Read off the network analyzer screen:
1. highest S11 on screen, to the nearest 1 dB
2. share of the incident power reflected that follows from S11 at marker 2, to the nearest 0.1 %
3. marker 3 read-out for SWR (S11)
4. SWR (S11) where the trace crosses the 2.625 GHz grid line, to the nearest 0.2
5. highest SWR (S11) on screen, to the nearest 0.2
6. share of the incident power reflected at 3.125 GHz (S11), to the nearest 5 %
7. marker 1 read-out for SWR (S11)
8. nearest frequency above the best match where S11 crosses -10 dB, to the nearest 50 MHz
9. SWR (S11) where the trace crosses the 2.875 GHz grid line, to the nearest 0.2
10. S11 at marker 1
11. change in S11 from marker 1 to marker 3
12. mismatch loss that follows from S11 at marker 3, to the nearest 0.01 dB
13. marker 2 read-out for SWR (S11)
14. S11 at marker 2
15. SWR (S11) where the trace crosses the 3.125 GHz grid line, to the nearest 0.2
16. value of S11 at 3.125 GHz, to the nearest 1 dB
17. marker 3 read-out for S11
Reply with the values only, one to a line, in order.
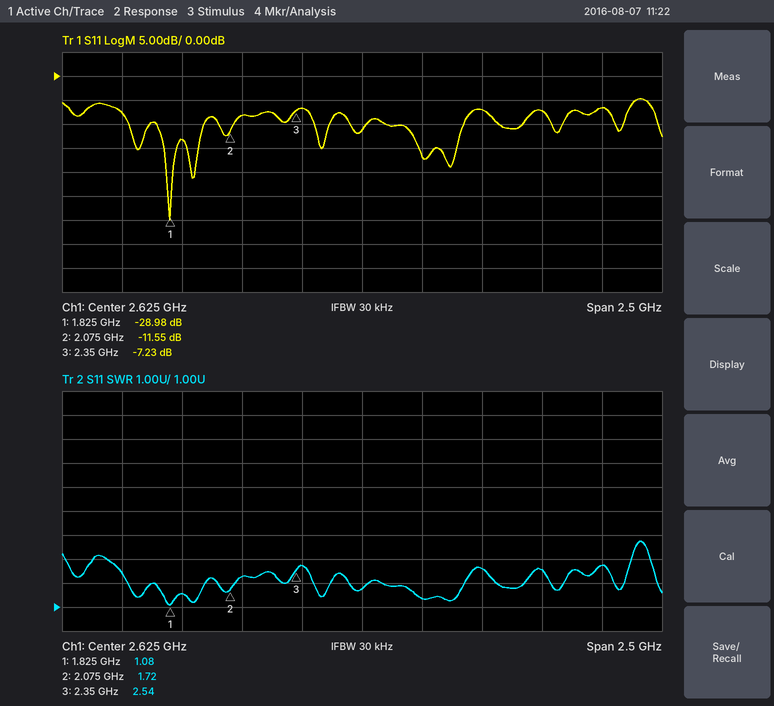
-5 dB
7.0 %
2.54
1.8
3.8
20 %
1.08
1.95 GHz
1.4
-28.98 dB
21.75 dB
0.91 dB
1.72
-11.55 dB
2.6
-7 dB
-7.23 dB
